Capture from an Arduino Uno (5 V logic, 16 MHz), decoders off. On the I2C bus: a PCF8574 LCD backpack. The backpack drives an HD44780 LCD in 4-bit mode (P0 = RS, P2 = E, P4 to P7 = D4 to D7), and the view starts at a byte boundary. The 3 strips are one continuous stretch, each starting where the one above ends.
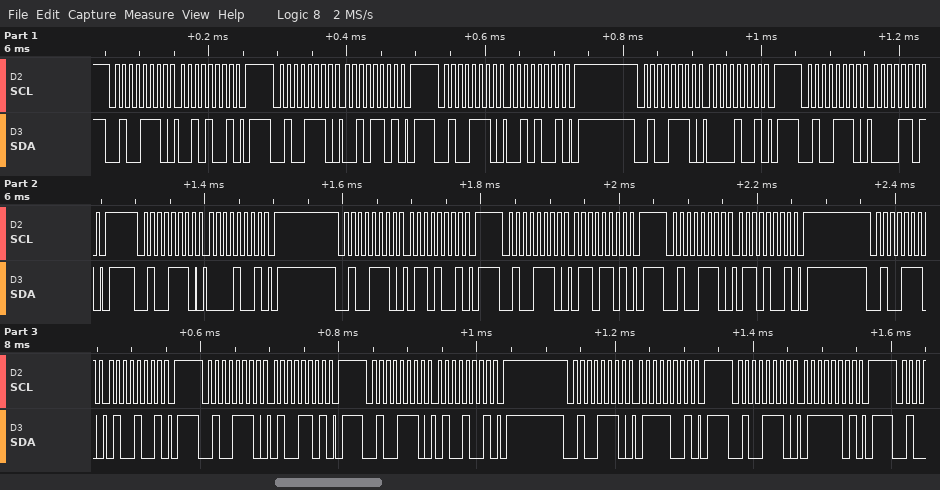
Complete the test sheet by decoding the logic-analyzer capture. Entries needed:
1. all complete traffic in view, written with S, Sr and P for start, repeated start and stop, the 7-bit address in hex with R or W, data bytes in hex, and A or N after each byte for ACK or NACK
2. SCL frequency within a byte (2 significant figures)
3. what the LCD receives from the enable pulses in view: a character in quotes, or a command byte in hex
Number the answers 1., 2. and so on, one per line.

1. S 27W A 29 A P S 27W A 2D A P S 27W A 29 A P S 27W A 09 A P S 27W A 0D A P S 27W A 09 A P S 27W A 69 A P S 27W A 6D A P S 27W A 69 A P S 27W A 49 A P S 27W A 4D A P S 27W A 49 A P S 27W A 79 A P S 27W A 7D A P
2. 100 kHz
3. ' ' 'd'
